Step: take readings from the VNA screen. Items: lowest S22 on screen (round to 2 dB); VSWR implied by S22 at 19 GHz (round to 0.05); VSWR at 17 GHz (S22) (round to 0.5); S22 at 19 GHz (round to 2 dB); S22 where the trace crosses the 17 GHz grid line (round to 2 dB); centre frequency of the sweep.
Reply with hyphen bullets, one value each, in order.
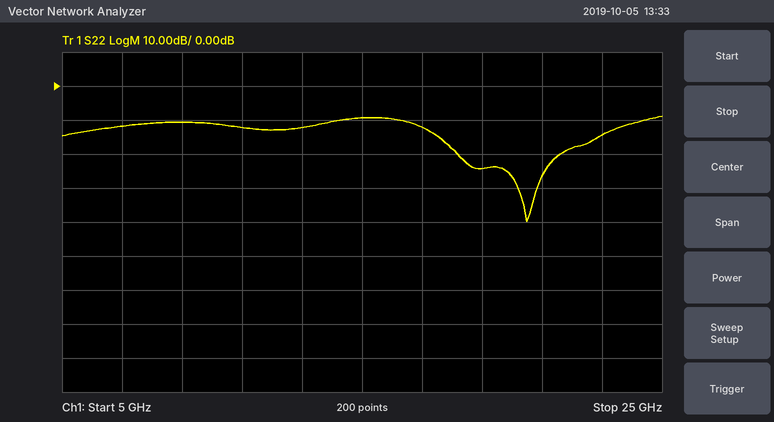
- -40 dB
- 1.15
- 1.5
- -24 dB
- -12 dB
- 15 GHz
